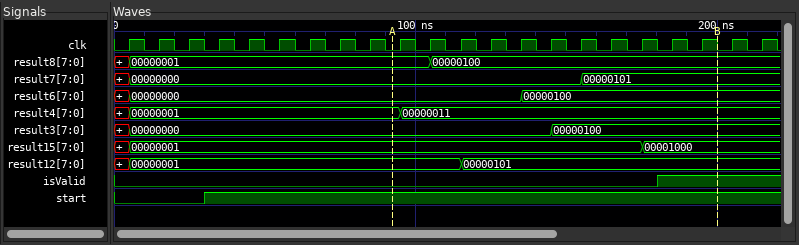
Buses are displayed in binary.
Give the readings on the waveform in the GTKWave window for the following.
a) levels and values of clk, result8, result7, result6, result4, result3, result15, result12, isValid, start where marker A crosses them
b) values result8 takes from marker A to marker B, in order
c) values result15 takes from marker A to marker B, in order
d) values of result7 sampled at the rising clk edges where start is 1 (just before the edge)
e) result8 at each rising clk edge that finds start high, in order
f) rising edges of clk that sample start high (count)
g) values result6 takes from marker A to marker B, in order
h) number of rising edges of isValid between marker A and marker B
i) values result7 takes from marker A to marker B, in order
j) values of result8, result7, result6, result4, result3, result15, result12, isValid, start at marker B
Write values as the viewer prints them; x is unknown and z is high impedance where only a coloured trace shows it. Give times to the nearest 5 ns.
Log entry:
clk=0, result8=00000001, result7=00000000, result6=00000000, result4=00000001, result3=00000000, result15=00000001, result12=00000001, isValid=0, start=1
00000001, 00000100
00000001, 00001000
00000000, 00000000, 00000000, 00000000, 00000000, 00000000, 00000000, 00000000, 00000000, 00000000, 00000000, 00000000, 00000000, 00000101, 00000101, 00000101, 00000101, 00000101, 00000101
00000001, 00000001, 00000001, 00000001, 00000001, 00000001, 00000001, 00000001, 00000100, 00000100, 00000100, 00000100, 00000100, 00000100, 00000100, 00000100, 00000100, 00000100, 00000100
19
00000000, 00000100
1
00000000, 00000101
result8=00000100, result7=00000101, result6=00000100, result4=00000011, result3=00000100, result15=00001000, result12=00000101, isValid=1, start=1
